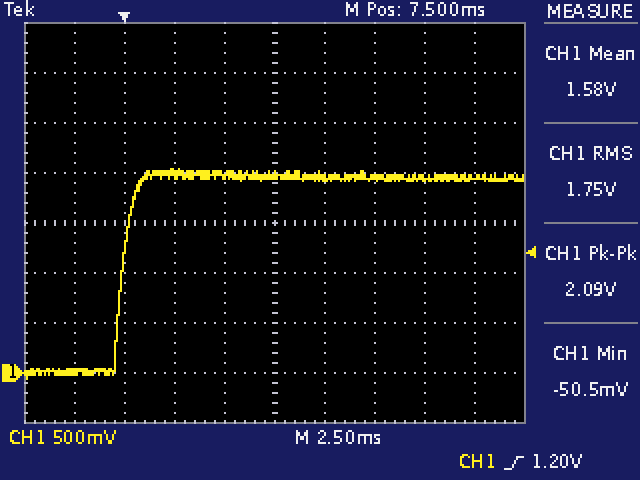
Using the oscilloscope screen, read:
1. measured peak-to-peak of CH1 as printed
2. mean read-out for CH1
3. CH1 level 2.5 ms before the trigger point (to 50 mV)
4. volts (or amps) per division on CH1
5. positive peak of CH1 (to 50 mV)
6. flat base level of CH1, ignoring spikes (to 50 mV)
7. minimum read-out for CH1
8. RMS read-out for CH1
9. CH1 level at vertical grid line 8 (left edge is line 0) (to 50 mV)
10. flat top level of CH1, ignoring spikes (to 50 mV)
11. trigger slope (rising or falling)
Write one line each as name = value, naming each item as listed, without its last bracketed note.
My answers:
measured peak-to-peak of CH1 as printed = 2.09 V
mean read-out for CH1 = 1.58 V
CH1 level 2.5 ms before the trigger point = 0 mV
volts (or amps) per division on CH1 = 500 mV
positive peak of CH1 = 2.05 V
flat base level of CH1, ignoring spikes = 0 mV
minimum read-out for CH1 = -50.5 mV
RMS read-out for CH1 = 1.75 V
CH1 level at vertical grid line 8 (left edge is line 0) = 1.95 V
flat top level of CH1, ignoring spikes = 1.95 V
trigger slope = rising
